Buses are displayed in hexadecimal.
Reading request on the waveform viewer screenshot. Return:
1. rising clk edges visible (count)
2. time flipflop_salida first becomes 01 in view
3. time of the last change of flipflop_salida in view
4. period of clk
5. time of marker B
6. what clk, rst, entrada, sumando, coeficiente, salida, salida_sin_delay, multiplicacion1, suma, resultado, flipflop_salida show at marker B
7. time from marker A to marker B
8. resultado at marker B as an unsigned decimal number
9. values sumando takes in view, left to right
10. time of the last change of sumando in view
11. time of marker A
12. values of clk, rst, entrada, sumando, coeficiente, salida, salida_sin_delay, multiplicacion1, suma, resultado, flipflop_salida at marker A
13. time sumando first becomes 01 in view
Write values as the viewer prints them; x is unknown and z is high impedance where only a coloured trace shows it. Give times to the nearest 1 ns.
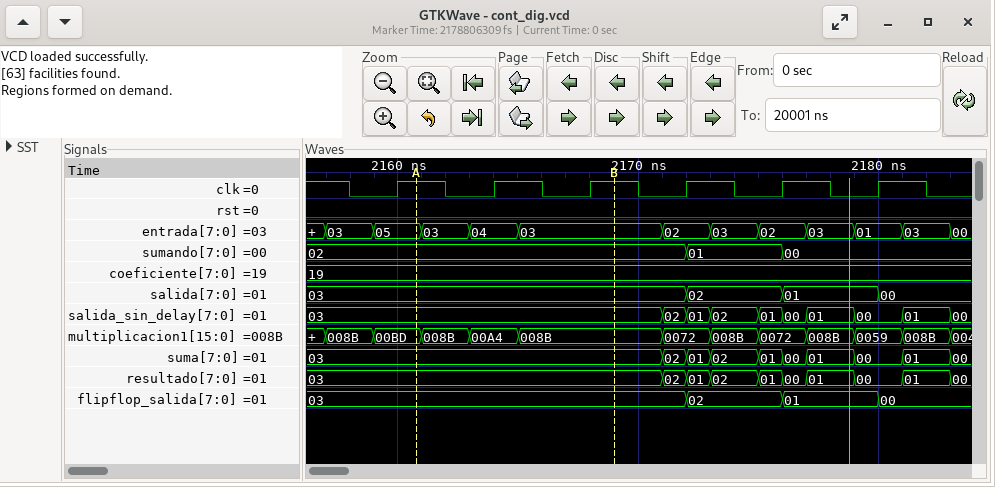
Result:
6
2176 ns
2180 ns
4 ns
2169 ns
clk=1, rst=0, entrada=03, sumando=02, coeficiente=19, salida=03, salida_sin_delay=03, multiplicacion1=008B, suma=03, resultado=03, flipflop_salida=03
8 ns
3
02, 01, 00
2176 ns
2161 ns
clk=1, rst=0, entrada=05, sumando=02, coeficiente=19, salida=03, salida_sin_delay=03, multiplicacion1=00BD, suma=03, resultado=03, flipflop_salida=03
2172 ns
